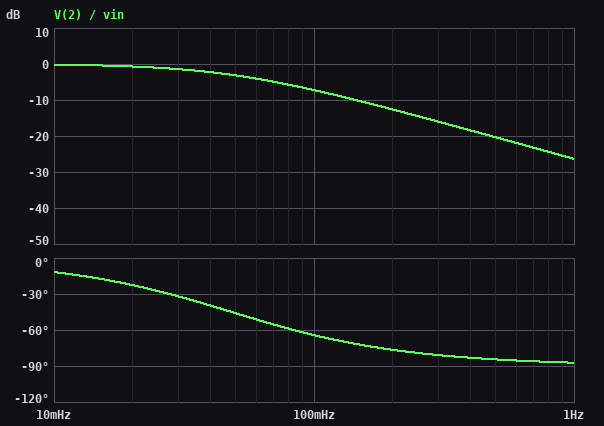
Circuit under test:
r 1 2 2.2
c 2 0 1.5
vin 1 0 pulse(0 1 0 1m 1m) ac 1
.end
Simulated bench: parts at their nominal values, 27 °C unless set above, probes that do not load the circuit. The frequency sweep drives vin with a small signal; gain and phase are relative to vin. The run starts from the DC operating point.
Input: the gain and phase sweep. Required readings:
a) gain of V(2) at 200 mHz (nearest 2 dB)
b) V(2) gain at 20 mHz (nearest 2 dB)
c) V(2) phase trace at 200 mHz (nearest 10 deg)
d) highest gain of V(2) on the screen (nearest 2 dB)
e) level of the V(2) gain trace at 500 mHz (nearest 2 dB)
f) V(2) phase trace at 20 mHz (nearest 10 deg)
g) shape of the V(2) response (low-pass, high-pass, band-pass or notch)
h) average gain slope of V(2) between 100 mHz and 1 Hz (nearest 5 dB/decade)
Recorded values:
-12 dB
0 dB
-80 deg
0 dB
-20 dB
-20 deg
low-pass
-20 dB/decade
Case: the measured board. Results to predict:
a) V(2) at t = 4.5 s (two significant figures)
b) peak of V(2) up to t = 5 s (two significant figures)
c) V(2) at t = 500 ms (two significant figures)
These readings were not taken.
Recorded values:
740 mV
780 mV
140 mV
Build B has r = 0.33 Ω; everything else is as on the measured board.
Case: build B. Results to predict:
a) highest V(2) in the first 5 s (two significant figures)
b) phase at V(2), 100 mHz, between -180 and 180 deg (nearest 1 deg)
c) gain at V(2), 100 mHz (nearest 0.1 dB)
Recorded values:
1.0 V
-17 deg
-0.4 dB
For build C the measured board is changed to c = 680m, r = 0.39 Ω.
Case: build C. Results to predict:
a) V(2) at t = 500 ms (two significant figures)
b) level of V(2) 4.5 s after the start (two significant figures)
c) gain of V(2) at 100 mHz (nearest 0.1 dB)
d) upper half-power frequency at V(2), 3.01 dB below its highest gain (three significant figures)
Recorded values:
850 mV
1.0 V
-0.1 dB
600 mHz
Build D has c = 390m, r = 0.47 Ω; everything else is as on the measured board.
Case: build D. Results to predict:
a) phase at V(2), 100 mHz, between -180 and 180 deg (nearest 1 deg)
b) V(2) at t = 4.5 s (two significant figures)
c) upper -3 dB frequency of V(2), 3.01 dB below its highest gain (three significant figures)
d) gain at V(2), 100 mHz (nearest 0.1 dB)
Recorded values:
-7 deg
1.0 V
868 mHz
-0.1 dB
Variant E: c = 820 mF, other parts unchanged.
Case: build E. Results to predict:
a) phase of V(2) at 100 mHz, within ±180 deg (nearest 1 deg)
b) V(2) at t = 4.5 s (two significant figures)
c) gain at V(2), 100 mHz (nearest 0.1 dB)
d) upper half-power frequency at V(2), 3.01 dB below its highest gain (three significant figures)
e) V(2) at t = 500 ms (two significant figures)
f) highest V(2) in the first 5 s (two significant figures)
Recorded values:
-49 deg
920 mV
-3.6 dB
88.2 mHz
240 mV
940 mV
